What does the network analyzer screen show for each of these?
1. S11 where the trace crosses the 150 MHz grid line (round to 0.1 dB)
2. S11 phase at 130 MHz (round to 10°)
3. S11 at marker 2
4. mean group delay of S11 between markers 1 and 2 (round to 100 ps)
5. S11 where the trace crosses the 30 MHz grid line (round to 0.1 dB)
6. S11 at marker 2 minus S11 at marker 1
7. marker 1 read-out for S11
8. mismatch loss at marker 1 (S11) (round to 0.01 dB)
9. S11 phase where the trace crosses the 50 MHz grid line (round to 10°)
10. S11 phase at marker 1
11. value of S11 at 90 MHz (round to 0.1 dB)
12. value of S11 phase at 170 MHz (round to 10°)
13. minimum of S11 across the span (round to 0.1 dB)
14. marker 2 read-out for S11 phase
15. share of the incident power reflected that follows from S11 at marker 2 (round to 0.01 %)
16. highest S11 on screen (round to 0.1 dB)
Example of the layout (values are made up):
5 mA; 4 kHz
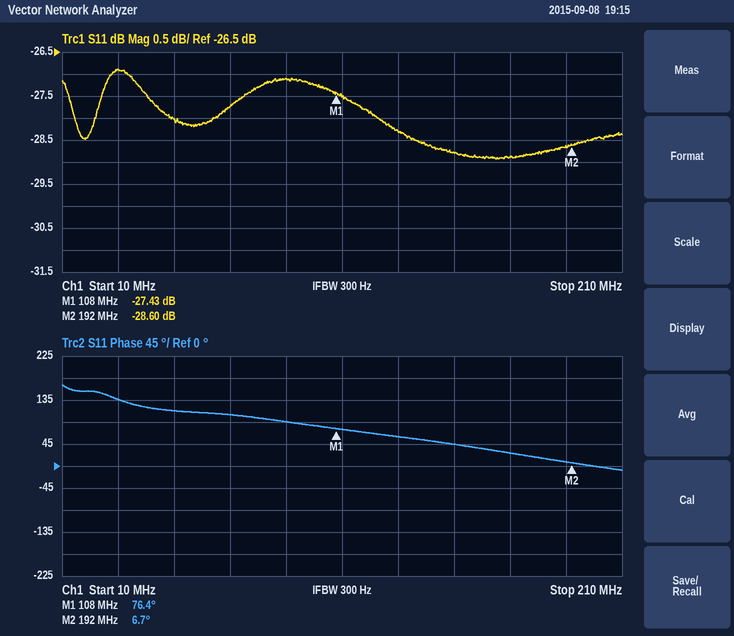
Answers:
-28.8 dB; 60°; -28.60 dB; 2.3 ns; -26.9 dB; -1.17 dB; -27.43 dB; 0.01 dB; 110°; 76.4°; -27.1 dB; 30°; -28.9 dB; 6.7°; 0.14 %; -26.9 dB
